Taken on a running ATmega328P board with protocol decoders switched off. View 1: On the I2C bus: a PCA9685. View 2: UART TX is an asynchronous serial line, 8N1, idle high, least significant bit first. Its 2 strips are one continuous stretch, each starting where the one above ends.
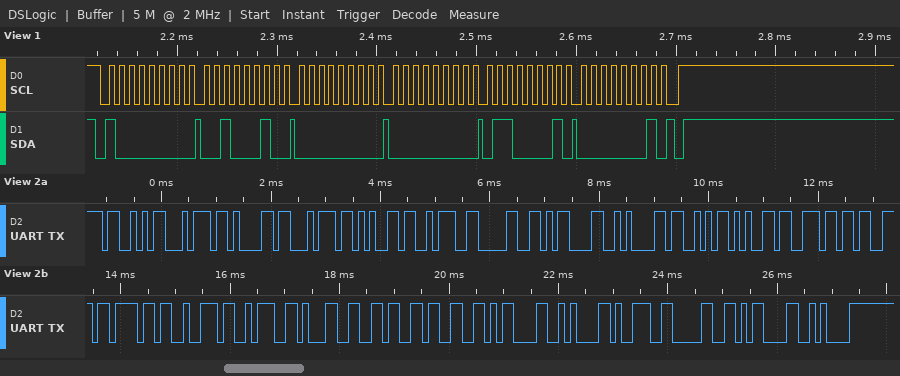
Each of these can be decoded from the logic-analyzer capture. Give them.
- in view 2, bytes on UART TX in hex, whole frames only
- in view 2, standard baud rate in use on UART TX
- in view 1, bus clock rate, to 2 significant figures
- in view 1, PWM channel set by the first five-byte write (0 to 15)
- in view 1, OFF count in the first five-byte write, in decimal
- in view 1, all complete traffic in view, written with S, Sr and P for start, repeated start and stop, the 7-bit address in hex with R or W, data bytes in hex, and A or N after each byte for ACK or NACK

53 74 61 74 65 3A 30 0D 0A 53 65 6E 73 6F 72 3A 31 36 33 0D 0A 39 30 0D 0A
9600 baud
100 kHz
7
353
S 40W A 22 A 00 A 00 A 61 A 01 A P
